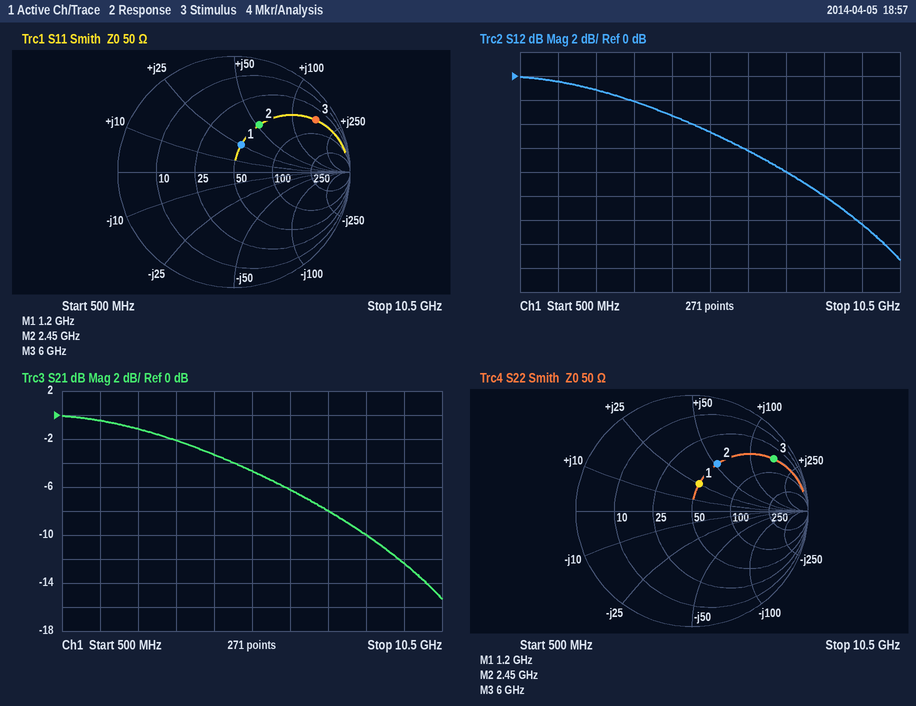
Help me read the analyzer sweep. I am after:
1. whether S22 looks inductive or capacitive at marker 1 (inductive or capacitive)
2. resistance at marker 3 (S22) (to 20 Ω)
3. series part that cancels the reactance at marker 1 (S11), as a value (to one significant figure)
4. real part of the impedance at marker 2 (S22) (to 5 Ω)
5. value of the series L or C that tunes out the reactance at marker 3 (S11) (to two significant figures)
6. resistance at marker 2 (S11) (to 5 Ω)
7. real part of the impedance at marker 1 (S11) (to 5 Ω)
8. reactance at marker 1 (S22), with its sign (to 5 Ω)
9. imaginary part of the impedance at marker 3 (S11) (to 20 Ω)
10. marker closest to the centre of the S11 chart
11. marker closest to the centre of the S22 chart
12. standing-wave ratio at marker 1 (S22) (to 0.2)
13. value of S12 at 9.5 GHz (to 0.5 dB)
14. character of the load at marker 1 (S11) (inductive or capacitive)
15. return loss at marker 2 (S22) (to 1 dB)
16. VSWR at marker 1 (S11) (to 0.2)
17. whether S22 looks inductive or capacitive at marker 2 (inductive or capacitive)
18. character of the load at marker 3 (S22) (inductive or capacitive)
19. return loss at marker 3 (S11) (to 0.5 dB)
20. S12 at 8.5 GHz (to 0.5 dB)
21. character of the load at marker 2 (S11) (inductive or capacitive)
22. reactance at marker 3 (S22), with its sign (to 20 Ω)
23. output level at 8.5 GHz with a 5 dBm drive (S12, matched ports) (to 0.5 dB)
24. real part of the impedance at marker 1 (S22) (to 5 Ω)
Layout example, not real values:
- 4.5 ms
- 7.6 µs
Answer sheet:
- inductive
- 60 Ω
- 5 pF
- 50 Ω
- 170 fF
- 50 Ω
- 50 Ω
- +25 Ω
- +160 Ω
- marker 1
- marker 1
- 1.6
- -12.5 dB
- inductive
- 7 dB
- 1.6
- inductive
- inductive
- 1.5 dB
- -10.0 dB
- inductive
- +160 Ω
- -5.0 dBm
- 50 Ω
